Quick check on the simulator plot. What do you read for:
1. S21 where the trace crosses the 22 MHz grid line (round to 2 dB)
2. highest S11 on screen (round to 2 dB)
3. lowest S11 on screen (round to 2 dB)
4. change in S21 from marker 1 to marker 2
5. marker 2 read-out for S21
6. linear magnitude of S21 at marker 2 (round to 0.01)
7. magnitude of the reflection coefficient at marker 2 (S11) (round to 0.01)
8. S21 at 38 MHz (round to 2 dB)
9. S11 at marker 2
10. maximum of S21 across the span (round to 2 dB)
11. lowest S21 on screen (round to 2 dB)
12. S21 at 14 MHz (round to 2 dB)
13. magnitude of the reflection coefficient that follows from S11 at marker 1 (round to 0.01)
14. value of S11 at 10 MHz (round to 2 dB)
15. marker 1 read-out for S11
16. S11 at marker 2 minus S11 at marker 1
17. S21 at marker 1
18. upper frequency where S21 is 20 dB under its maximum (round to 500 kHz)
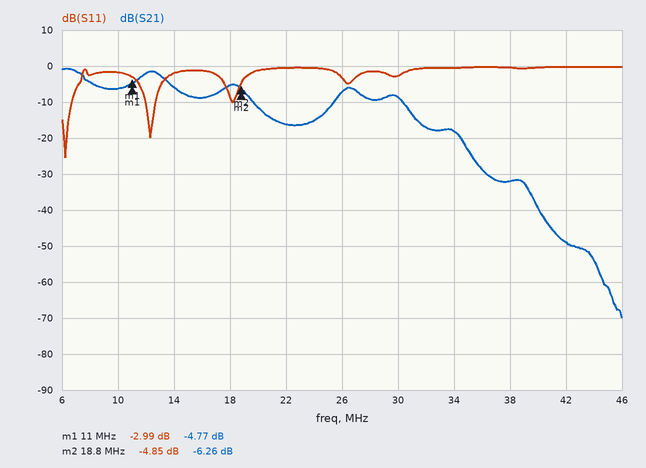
-16 dB
0 dB
-26 dB
-1.49 dB
-6.26 dB
0.49
0.57
-32 dB
-4.85 dB
0 dB
-70 dB
-6 dB
0.71
-2 dB
-2.99 dB
-1.86 dB
-4.77 dB
34.5 MHz
